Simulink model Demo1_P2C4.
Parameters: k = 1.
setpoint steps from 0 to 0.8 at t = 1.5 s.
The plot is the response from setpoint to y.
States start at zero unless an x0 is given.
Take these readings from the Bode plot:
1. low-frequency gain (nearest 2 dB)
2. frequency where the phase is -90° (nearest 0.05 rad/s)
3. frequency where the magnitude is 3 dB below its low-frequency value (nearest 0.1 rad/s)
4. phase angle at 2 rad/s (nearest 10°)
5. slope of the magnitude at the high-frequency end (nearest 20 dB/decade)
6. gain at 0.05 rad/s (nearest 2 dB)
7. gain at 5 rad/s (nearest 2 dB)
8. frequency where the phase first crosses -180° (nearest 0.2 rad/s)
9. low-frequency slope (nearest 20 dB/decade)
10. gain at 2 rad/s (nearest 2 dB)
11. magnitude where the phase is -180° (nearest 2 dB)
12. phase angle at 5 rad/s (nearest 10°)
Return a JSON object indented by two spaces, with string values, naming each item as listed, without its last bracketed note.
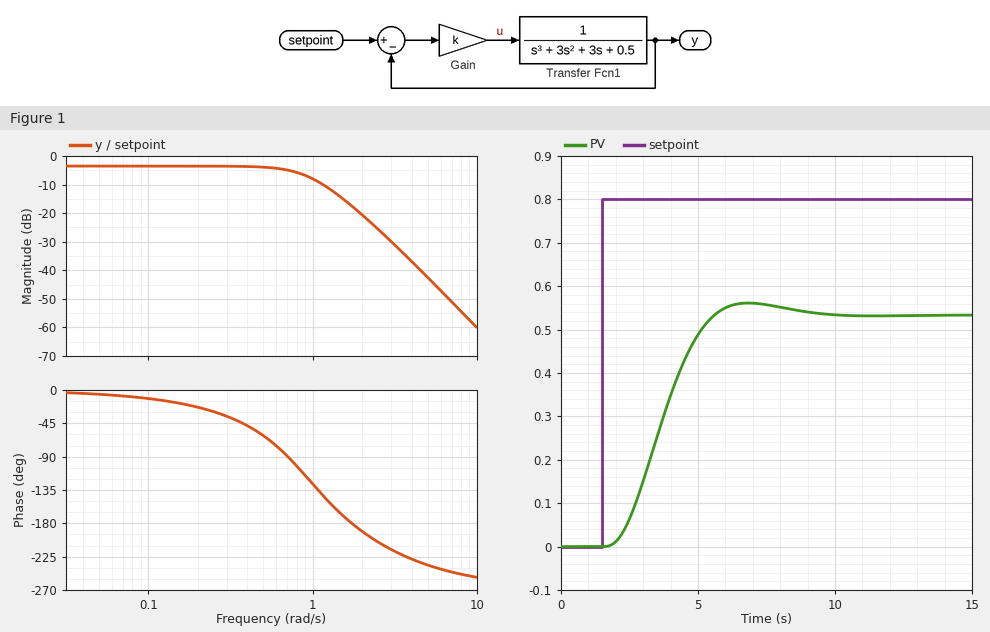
{
  "low-frequency gain": "-4 dB",
  "frequency where the phase is -90°": "0.70 rad/s",
  "frequency where the magnitude is 3 dB below its low-frequency value": "0.9 rad/s",
  "phase angle at 2 rad/s": "-190°",
  "slope of the magnitude at the high-frequency end": "-60 dB/decade",
  "gain at 0.05 rad/s": "-4 dB",
  "gain at 5 rad/s": "-42 dB",
  "frequency where the phase first crosses -180°": "1.8 rad/s",
  "low-frequency slope": "0 dB/decade",
  "gain at 2 rad/s": "-20 dB",
  "magnitude where the phase is -180°": "-18 dB",
  "phase angle at 5 rad/s": "-240°"
}
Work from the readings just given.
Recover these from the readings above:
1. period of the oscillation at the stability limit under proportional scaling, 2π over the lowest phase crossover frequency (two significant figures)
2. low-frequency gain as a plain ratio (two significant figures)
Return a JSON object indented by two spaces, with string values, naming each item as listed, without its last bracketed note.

{
  "period of the oscillation at the stability limit under proportional scaling, 2π over the lowest phase crossover frequency": "3.5 s",
  "low-frequency gain as a plain ratio": "0.63"
}
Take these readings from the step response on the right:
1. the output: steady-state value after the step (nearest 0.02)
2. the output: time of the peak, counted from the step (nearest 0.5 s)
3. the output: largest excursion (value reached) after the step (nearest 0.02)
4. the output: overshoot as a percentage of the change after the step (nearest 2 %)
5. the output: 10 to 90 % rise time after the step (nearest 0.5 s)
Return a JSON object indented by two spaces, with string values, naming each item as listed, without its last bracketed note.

{
  "the output: steady-state value after the step": "0.54",
  "the output: time of the peak, counted from the step": "5.5 s",
  "the output: largest excursion (value reached) after the step": "0.56",
  "the output: overshoot as a percentage of the change after the step": "6 %",
  "the output: 10 to 90 % rise time after the step": "2.5 s"
}
